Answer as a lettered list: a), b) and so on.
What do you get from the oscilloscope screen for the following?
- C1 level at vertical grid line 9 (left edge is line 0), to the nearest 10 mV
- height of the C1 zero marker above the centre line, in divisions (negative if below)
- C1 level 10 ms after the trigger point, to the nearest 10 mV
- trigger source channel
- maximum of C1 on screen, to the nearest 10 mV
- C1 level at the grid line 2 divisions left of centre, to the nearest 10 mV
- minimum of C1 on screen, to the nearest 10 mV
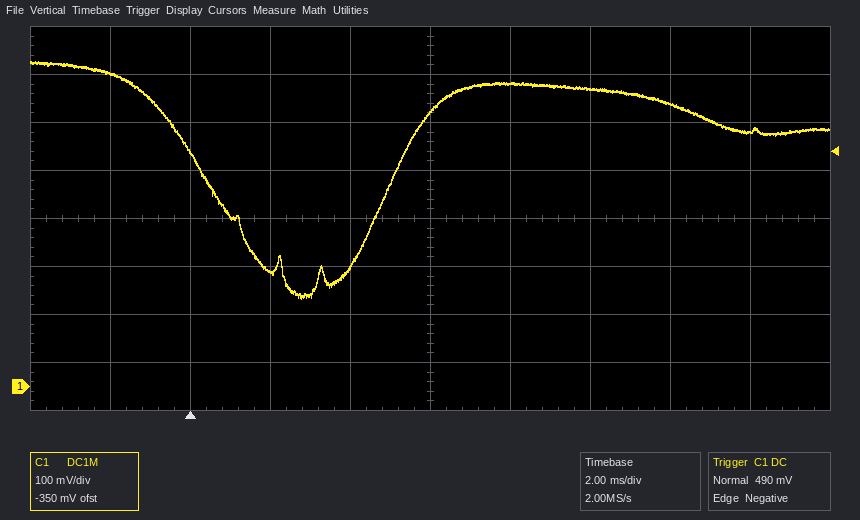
a) 530 mV
b) -3.5 div
c) 620 mV
d) C1
e) 680 mV
f) 240 mV
g) 180 mV
